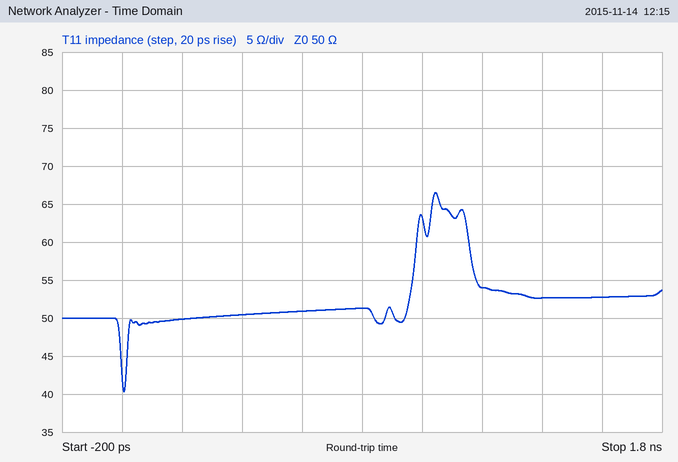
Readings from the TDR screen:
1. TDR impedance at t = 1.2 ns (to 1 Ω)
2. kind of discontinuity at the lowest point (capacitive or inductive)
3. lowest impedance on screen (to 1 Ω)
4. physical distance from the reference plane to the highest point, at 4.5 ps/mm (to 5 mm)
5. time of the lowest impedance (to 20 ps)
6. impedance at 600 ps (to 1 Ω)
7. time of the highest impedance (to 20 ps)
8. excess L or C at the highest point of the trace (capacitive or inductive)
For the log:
54 Ω
capacitive
40 Ω
115 mm
0 ps
51 Ω
1.04 ns
inductive
